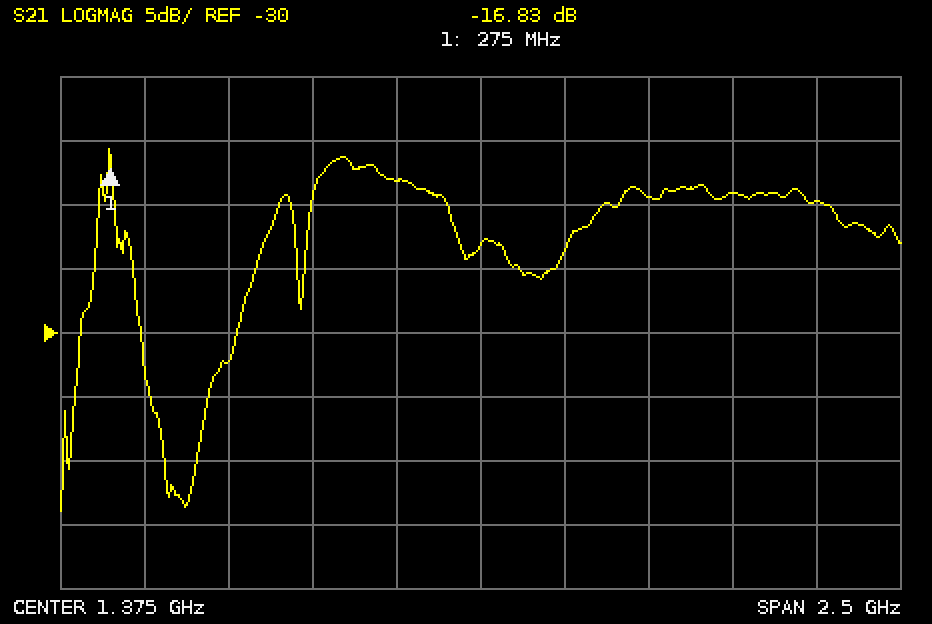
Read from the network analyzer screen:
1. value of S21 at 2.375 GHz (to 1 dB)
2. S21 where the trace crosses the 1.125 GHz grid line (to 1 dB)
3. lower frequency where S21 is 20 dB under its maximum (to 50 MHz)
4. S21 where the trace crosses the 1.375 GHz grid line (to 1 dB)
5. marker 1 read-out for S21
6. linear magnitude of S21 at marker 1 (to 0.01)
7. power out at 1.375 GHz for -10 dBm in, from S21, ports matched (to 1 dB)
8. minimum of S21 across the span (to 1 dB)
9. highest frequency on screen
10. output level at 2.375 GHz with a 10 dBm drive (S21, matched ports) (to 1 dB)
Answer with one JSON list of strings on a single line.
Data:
["-20 dB", "-18 dB", "150 MHz", "-23 dB", "-16.83 dB", "0.14", "-33 dBm", "-44 dB", "2.625 GHz", "-10 dBm"]
